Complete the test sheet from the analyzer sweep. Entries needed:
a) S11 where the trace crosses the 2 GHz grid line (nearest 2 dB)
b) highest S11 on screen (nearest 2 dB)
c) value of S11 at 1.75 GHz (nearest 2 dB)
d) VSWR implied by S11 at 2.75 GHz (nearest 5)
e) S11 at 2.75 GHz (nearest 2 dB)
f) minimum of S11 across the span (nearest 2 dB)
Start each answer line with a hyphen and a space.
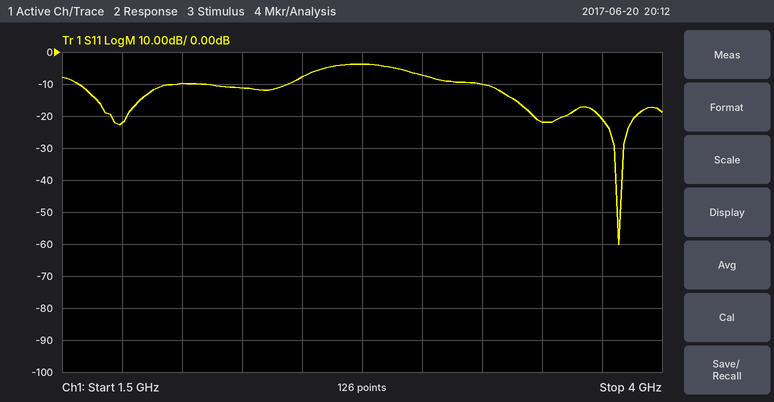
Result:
- -10 dB
- -4 dB
- -22 dB
- 5
- -4 dB
- -60 dB
